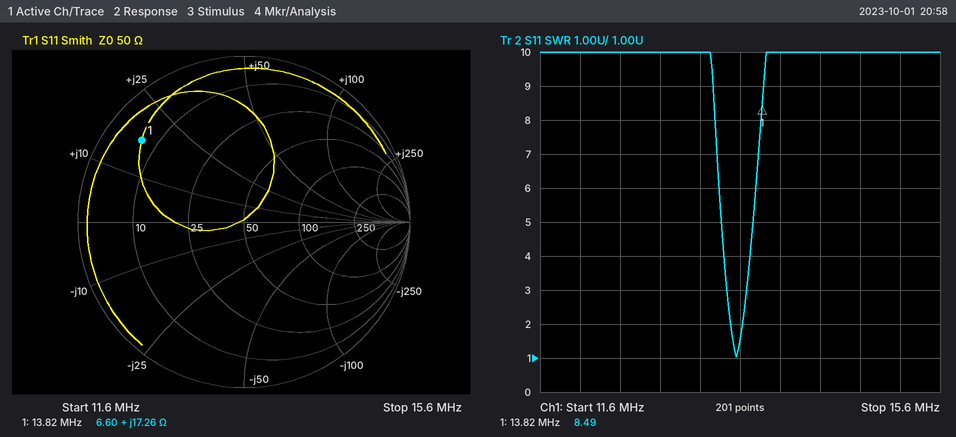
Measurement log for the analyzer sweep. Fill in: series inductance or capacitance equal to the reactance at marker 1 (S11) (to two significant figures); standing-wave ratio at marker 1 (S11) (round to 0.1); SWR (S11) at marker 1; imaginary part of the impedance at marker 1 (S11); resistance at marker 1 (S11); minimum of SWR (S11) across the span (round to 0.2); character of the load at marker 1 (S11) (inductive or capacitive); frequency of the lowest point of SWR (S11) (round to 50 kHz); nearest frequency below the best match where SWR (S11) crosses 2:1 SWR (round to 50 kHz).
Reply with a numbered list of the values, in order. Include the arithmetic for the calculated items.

1. L = 17.26 Ω/(2π × 13.82 MHz) ≈ 199 nH, so 200 nH to two significant figures
2. 8.5
3. 8.49
4. +17.26 Ω
5. 6.60 Ω
6. 1.0
7. inductive
8. 13.55 MHz
9. 13.50 MHz
